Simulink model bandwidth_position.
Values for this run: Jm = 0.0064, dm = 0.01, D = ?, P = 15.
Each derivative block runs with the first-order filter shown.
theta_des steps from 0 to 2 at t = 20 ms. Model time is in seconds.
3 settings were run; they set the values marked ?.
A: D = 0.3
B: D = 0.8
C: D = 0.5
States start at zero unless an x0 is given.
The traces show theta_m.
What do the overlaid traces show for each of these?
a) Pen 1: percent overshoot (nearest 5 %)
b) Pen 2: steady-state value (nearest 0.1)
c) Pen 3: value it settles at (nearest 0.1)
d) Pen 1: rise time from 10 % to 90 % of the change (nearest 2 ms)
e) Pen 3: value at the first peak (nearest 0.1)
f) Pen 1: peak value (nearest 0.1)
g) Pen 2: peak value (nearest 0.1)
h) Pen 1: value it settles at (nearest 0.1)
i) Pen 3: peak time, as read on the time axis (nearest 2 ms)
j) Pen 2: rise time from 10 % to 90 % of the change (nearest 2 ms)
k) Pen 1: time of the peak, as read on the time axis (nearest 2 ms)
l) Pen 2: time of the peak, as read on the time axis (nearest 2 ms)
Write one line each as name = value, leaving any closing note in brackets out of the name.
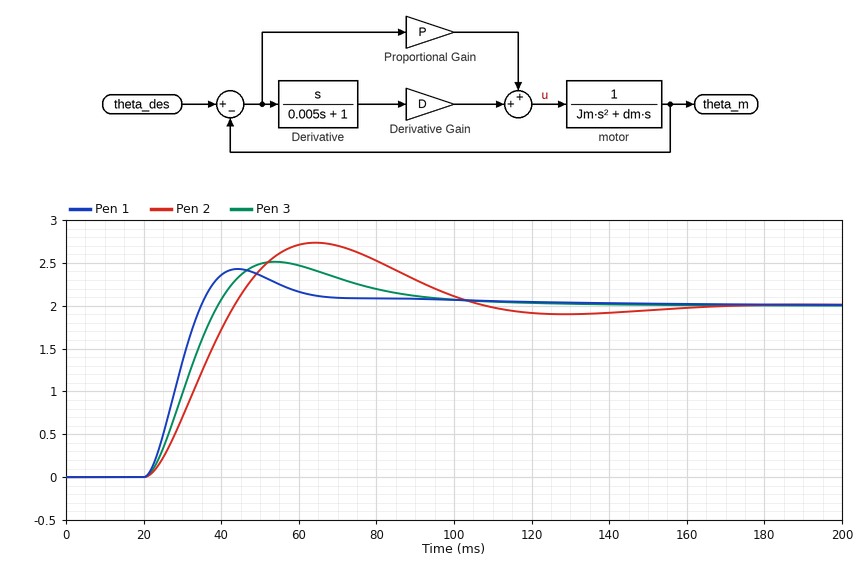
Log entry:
Pen 1: percent overshoot = 20 %
Pen 2: steady-state value = 2.0
Pen 3: value it settles at = 2.0
Pen 1: rise time from 10 % to 90 % of the change = 10 ms
Pen 3: value at the first peak = 2.5
Pen 1: peak value = 2.4
Pen 2: peak value = 2.7
Pen 1: value it settles at = 2.0
Pen 3: peak time, as read on the time axis = 54 ms
Pen 2: rise time from 10 % to 90 % of the change = 16 ms
Pen 1: time of the peak, as read on the time axis = 44 ms
Pen 2: time of the peak, as read on the time axis = 64 ms
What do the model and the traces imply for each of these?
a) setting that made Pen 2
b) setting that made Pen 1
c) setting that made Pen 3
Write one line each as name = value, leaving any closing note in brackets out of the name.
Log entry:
setting that made Pen 2 = A
setting that made Pen 1 = B
setting that made Pen 3 = C
